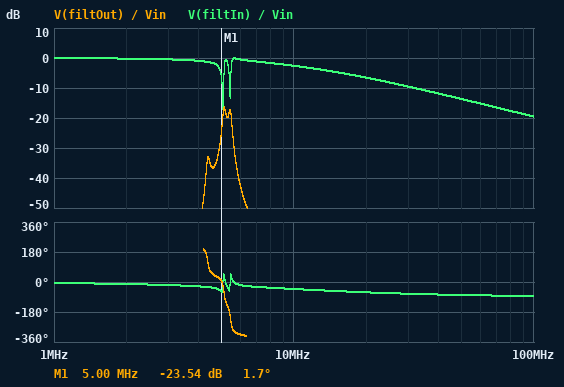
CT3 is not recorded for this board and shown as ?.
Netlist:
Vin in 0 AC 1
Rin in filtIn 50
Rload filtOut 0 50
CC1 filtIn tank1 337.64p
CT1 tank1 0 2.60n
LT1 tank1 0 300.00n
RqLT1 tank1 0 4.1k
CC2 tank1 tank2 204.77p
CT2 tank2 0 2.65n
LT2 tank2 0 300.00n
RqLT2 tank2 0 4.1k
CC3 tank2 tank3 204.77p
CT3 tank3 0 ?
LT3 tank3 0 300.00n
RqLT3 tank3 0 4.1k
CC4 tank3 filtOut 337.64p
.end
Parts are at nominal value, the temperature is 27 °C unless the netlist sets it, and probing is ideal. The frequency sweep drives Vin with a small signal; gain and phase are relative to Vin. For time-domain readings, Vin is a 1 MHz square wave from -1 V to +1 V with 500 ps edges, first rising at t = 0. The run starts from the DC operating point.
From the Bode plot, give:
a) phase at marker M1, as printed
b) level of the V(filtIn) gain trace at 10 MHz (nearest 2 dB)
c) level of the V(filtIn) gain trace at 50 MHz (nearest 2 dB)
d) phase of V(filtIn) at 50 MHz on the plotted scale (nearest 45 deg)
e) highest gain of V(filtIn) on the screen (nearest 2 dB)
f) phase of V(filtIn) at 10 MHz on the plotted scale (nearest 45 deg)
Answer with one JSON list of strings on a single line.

["1.7 deg", "-2 dB", "-14 dB", "-90 deg", "0 dB", "-45 deg"]
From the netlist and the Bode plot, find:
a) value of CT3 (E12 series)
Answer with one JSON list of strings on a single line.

["3.9 nF"]
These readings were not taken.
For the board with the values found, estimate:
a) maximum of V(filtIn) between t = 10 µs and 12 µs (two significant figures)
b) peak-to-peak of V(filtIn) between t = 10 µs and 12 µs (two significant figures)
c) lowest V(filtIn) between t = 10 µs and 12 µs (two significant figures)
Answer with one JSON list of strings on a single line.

["1.2 V", "2.3 V", "-1.2 V"]
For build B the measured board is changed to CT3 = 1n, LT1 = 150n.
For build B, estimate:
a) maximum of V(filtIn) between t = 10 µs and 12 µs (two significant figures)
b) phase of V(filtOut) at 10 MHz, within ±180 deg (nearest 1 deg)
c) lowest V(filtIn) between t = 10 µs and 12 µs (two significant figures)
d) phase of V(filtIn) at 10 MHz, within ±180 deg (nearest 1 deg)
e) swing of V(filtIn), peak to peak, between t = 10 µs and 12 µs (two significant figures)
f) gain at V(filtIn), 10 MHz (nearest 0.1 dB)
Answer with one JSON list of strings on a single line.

["1.1 V", "24 deg", "-1.1 V", "-39 deg", "2.2 V", "-2.2 dB"]
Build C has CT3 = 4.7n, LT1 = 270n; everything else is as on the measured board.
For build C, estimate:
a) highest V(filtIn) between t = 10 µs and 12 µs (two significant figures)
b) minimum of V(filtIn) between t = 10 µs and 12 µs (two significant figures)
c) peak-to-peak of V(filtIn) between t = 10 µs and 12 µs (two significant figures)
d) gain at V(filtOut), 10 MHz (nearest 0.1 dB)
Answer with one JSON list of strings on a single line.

["1.1 V", "-1.1 V", "2.2 V", "-68.5 dB"]
